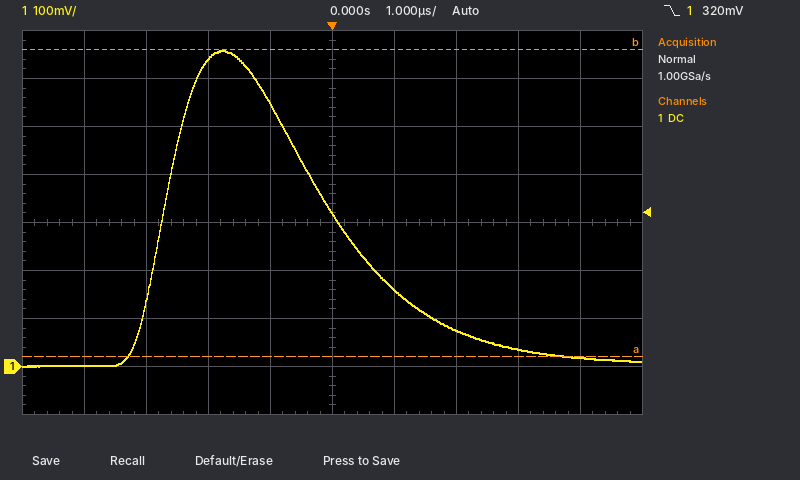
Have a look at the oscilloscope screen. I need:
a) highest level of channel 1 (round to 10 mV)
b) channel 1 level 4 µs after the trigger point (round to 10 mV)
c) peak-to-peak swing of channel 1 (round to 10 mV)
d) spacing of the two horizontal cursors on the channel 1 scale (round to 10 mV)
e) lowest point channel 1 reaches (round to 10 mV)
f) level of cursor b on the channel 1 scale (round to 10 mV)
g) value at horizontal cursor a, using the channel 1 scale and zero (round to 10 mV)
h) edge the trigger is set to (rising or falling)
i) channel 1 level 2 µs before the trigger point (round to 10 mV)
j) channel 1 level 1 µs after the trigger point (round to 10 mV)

660 mV
20 mV
660 mV
640 mV
0 mV
660 mV
20 mV
falling
640 mV
160 mV
